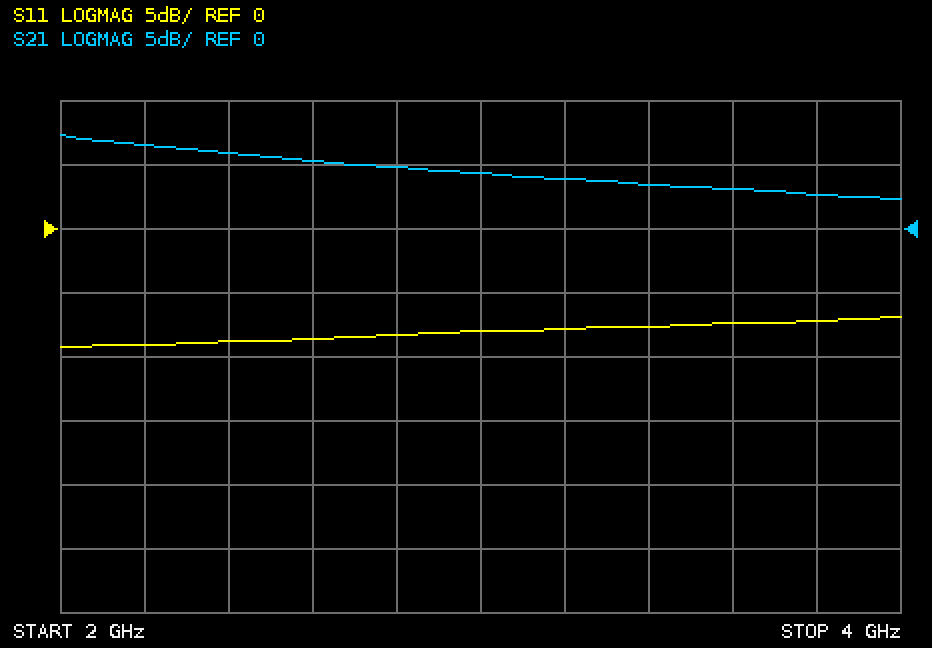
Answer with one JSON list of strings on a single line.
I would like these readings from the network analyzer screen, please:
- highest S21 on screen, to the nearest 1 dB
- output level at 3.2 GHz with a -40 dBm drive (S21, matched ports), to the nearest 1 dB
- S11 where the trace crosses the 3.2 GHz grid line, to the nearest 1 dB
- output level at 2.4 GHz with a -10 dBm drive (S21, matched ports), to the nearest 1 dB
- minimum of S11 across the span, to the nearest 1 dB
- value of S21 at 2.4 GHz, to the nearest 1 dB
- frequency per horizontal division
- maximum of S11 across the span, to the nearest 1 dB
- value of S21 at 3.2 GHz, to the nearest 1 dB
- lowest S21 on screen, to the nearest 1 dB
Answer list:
["7 dB", "-36 dBm", "-8 dB", "-4 dBm", "-9 dB", "6 dB", "200 MHz", "-7 dB", "4 dB", "2 dB"]
